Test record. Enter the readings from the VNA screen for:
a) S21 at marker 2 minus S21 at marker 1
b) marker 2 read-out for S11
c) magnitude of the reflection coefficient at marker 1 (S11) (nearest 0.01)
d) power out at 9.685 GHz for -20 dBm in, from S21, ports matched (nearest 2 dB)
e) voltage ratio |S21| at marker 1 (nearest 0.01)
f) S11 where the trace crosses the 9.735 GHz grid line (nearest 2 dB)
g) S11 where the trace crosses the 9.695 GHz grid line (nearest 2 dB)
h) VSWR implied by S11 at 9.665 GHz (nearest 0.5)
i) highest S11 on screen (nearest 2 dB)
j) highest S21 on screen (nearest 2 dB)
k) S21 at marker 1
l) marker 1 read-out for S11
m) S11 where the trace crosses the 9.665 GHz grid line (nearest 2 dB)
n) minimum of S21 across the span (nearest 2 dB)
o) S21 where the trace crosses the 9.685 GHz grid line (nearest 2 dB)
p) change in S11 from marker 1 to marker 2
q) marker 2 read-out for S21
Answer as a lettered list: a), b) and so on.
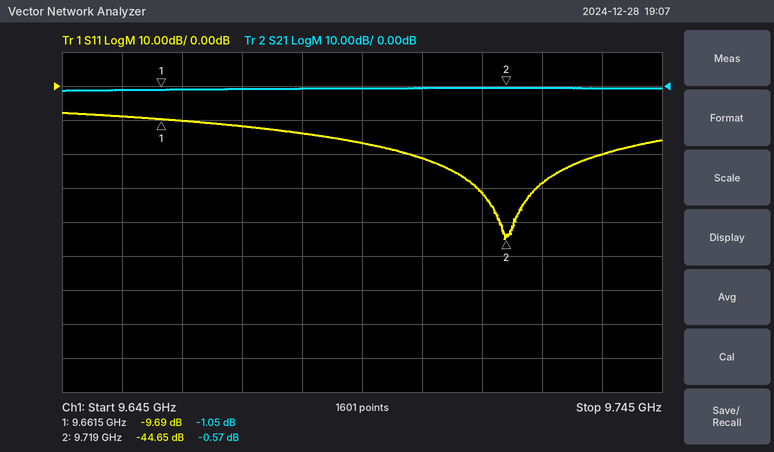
a) 0.48 dB
b) -44.65 dB
c) 0.33
d) -20 dBm
e) 0.89
f) -20 dB
g) -16 dB
h) 2.0
i) -8 dB
j) 0 dB
k) -1.05 dB
l) -9.69 dB
m) -10 dB
n) -2 dB
o) 0 dB
p) -34.96 dB
q) -0.57 dB
